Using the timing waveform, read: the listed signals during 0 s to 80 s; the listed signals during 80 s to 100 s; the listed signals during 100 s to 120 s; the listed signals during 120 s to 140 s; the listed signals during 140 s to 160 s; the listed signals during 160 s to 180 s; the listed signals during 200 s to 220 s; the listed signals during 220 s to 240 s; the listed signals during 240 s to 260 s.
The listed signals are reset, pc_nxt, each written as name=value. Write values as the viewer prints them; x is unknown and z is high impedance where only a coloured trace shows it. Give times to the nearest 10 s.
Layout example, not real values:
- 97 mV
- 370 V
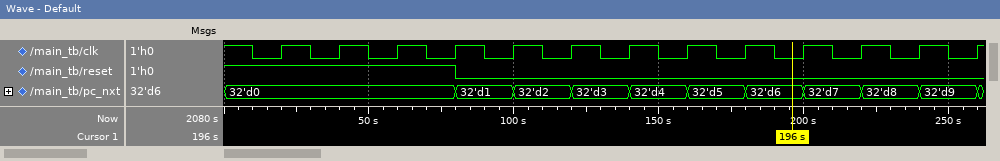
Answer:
- reset=1, pc_nxt=32'd0
- reset=0, pc_nxt=32'd1
- reset=0, pc_nxt=32'd2
- reset=0, pc_nxt=32'd3
- reset=0, pc_nxt=32'd4
- reset=0, pc_nxt=32'd5
- reset=0, pc_nxt=32'd7
- reset=0, pc_nxt=32'd8
- reset=0, pc_nxt=32'd9
